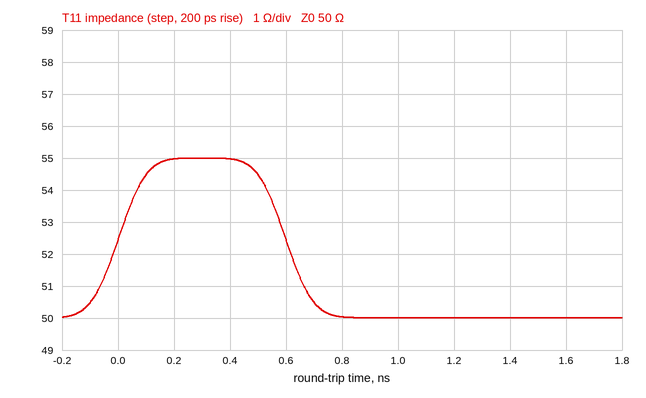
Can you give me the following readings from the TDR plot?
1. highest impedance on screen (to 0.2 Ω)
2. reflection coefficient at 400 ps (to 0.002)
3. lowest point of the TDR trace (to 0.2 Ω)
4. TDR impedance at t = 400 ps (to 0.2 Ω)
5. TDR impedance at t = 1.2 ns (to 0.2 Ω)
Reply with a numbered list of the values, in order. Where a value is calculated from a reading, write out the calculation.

1. 55.0 Ω
2. (55 − 50)/(55 + 50) ≈ +0.048
3. 50.0 Ω
4. 55.0 Ω
5. 50.0 Ω
